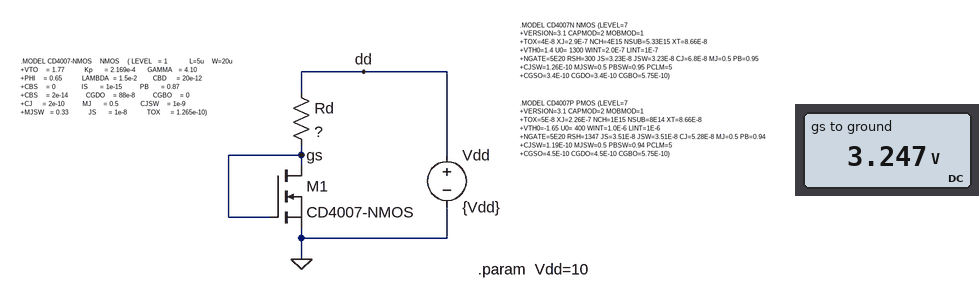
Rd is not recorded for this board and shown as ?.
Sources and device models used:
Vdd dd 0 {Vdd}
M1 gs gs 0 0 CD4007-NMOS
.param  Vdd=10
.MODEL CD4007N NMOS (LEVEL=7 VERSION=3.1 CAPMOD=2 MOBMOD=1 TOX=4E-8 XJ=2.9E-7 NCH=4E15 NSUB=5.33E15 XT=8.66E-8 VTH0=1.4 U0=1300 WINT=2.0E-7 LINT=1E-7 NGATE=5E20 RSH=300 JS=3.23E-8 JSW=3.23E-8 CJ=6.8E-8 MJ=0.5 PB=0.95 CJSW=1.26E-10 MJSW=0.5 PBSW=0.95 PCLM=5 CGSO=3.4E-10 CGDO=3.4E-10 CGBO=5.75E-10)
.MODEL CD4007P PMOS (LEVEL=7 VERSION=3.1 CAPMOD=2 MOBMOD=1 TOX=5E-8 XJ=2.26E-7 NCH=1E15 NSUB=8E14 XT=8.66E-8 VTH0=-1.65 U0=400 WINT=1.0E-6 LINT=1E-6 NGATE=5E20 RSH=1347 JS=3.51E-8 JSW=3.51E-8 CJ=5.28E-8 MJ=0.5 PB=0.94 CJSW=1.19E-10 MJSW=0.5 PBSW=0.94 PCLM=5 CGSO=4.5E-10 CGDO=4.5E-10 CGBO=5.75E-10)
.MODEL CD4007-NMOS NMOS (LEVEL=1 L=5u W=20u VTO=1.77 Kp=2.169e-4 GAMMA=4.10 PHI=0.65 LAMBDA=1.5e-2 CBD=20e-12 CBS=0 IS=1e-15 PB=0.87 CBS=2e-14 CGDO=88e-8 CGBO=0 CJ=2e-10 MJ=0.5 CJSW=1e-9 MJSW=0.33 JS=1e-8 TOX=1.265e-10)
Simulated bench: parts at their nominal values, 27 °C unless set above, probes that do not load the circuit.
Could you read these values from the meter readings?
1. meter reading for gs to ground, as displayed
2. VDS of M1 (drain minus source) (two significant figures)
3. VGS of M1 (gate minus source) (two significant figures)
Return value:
3.247 V
3.2 V
3.2 V
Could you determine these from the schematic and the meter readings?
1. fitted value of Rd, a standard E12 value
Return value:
6.8 kΩ
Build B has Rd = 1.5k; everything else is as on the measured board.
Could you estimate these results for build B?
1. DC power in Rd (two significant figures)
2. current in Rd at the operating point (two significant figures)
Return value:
20 mW
3.6 mA
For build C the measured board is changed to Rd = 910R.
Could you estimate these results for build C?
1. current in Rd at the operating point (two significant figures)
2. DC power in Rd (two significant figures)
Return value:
5.3 mA
26 mW
